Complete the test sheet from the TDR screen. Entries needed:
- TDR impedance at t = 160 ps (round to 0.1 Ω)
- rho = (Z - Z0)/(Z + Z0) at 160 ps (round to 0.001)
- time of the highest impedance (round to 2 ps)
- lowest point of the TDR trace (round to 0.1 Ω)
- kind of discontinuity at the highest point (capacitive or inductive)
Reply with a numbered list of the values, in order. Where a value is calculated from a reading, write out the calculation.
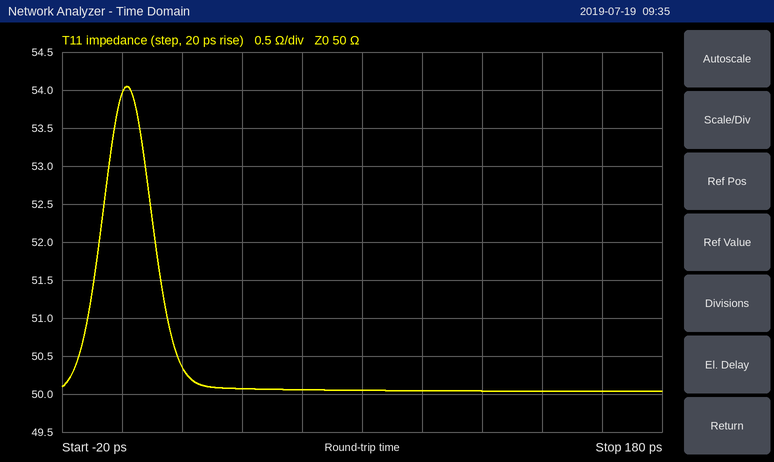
1. 50.0 Ω
2. (50 − 50)/(50 + 50) ≈ 0.000
3. 2 ps
4. 50.0 Ω
5. inductive
